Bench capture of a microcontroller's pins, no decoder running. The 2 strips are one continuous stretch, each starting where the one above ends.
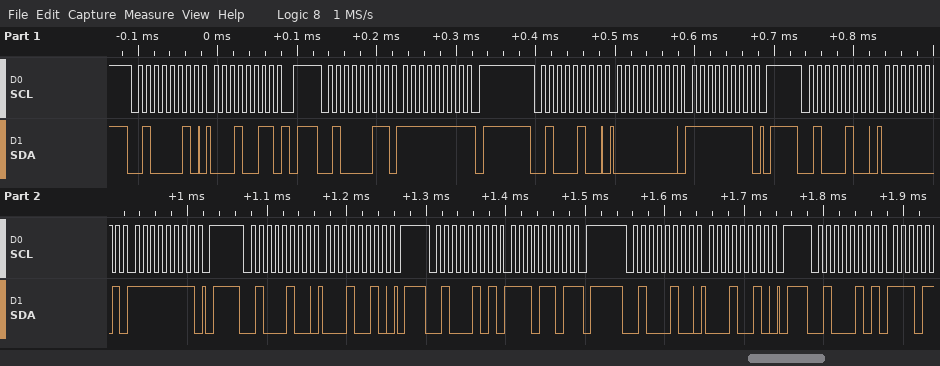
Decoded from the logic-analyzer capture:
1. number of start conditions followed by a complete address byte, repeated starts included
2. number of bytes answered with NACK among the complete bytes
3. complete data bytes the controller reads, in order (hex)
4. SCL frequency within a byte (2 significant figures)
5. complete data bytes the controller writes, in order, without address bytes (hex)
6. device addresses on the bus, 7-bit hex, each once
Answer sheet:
8
2
FF ED
100 kHz
13 00 FF 01 FF 12 12
0x21 0x22
